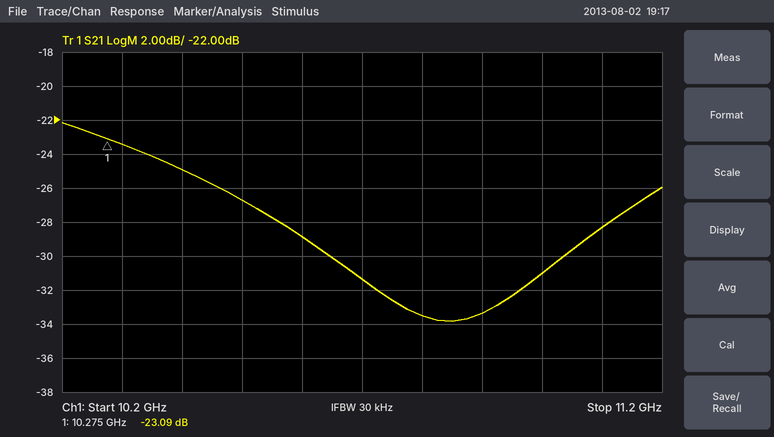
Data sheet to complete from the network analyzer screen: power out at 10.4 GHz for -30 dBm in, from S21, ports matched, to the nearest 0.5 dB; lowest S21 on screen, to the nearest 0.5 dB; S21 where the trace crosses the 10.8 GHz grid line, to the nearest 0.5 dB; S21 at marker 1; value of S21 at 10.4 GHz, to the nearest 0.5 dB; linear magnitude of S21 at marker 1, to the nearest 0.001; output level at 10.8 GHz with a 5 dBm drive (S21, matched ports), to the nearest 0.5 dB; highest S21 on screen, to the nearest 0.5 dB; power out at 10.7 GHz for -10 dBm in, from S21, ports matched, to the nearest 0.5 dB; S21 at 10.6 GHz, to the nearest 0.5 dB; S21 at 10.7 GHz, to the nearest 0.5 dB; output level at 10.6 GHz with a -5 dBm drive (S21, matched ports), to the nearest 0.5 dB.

-55.0 dBm
-34.0 dB
-33.5 dB
-23.09 dB
-25.0 dB
0.070
-28.5 dBm
-22.0 dB
-41.5 dBm
-29.0 dB
-31.5 dB
-34.0 dBm
